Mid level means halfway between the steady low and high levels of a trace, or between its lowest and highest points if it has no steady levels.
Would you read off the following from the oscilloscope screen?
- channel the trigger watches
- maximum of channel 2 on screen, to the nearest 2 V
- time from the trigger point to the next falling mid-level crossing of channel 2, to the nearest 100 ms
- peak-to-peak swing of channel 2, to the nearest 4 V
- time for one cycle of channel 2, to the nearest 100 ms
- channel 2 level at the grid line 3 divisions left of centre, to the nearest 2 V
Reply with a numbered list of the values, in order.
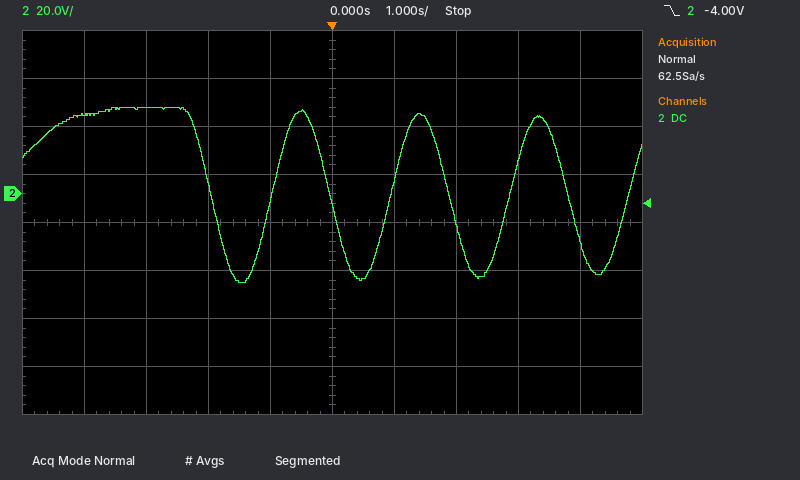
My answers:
1. channel 2
2. 36 V
3. 1.9 s
4. 72 V
5. 1.9 s
6. 36 V
